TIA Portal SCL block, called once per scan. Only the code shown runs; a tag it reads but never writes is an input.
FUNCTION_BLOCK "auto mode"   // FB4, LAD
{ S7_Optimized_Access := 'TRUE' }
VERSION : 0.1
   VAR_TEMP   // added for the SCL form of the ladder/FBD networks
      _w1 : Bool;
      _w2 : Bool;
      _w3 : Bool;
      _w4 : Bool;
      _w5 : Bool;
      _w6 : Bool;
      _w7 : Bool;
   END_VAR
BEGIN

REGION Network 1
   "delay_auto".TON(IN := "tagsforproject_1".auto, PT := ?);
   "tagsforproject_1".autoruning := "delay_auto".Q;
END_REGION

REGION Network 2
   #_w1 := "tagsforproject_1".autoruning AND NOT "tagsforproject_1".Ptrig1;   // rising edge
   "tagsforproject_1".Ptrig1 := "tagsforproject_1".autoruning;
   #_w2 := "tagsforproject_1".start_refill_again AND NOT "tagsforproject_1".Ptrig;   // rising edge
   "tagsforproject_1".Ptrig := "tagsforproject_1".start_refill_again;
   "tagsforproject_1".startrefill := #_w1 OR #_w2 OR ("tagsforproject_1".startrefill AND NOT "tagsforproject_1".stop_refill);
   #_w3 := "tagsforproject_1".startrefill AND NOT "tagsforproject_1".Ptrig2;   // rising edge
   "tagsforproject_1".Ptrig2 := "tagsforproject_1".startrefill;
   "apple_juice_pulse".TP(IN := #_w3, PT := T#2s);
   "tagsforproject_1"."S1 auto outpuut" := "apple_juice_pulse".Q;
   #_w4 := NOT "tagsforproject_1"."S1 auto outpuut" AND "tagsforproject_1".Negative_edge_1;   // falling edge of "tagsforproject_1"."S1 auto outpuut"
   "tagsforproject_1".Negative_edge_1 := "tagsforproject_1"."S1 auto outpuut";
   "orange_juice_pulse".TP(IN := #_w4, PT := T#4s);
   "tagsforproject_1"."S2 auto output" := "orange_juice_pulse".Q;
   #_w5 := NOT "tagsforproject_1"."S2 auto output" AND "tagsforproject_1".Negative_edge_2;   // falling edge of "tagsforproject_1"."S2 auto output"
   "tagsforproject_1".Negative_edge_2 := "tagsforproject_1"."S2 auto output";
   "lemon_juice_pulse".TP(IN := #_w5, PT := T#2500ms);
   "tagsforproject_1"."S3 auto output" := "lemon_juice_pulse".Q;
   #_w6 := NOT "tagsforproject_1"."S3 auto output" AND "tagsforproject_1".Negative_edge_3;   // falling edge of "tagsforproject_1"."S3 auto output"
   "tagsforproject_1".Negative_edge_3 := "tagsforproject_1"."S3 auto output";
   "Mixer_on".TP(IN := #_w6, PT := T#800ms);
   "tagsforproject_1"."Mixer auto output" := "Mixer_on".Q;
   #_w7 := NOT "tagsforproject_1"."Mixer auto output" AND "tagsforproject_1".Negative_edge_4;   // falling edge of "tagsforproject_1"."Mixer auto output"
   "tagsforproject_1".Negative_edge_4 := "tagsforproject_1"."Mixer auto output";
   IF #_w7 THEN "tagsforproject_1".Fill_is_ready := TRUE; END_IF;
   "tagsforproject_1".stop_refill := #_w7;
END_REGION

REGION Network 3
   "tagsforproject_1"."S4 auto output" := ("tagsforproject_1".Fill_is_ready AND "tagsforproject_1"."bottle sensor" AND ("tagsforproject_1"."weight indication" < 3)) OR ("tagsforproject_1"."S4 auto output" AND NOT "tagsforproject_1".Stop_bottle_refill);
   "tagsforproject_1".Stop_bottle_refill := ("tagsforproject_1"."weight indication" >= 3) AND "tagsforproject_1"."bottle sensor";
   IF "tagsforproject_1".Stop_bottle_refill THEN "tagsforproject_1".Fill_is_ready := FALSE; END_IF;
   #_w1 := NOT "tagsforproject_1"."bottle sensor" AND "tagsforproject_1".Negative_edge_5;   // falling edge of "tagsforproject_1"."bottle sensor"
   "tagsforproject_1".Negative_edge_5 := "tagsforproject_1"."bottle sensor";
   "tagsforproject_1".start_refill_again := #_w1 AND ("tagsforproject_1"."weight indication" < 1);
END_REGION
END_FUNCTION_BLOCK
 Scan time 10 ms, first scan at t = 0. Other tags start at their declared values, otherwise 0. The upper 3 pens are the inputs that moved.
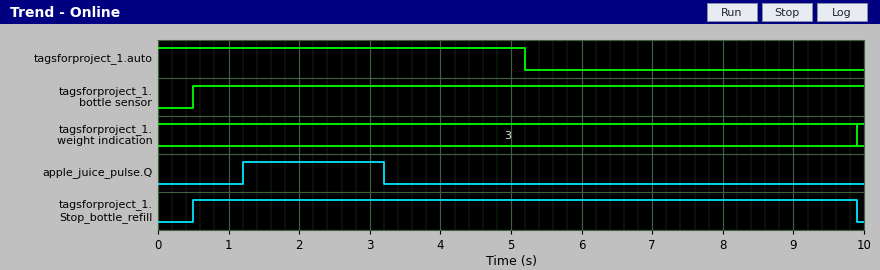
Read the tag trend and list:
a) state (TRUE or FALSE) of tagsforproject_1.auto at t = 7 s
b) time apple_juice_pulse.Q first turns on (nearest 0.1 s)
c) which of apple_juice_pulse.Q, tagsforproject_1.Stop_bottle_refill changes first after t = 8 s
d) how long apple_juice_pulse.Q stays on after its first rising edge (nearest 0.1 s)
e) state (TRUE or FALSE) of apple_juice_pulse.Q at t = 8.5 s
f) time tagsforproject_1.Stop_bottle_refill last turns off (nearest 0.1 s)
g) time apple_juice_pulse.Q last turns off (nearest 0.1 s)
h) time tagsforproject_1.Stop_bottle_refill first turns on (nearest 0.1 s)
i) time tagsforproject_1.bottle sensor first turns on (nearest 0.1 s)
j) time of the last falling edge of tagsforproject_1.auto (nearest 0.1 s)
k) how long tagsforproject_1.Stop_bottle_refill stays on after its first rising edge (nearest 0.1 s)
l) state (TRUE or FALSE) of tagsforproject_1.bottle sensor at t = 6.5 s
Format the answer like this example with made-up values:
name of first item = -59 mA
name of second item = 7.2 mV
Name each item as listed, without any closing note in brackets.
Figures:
state (TRUE or FALSE) of tagsforproject_1.auto at t = 7 s = FALSE
time apple_juice_pulse.Q first turns on = 1.2 s
which of apple_juice_pulse.Q, tagsforproject_1.Stop_bottle_refill changes first after t = 8 s = tagsforproject_1.Stop_bottle_refill
how long apple_juice_pulse.Q stays on after its first rising edge = 2.0 s
state (TRUE or FALSE) of apple_juice_pulse.Q at t = 8.5 s = FALSE
time tagsforproject_1.Stop_bottle_refill last turns off = 9.9 s
time apple_juice_pulse.Q last turns off = 3.2 s
time tagsforproject_1.Stop_bottle_refill first turns on = 0.5 s
time tagsforproject_1.bottle sensor first turns on = 0.5 s
time of the last falling edge of tagsforproject_1.auto = 5.2 s
how long tagsforproject_1.Stop_bottle_refill stays on after its first rising edge = 9.4 s
state (TRUE or FALSE) of tagsforproject_1.bottle sensor at t = 6.5 s = TRUE
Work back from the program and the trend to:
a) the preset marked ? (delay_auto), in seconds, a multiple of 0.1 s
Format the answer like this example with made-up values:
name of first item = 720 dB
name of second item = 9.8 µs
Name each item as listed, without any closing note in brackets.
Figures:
the preset marked ? (delay_auto), in seconds, a multiple of 0.1 s = 1.2 s
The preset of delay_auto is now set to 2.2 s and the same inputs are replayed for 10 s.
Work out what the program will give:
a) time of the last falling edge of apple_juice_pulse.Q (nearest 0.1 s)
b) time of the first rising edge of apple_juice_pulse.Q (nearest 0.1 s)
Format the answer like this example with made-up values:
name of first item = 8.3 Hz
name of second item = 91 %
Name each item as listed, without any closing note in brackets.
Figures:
time of the last falling edge of apple_juice_pulse.Q = 4.2 s
time of the first rising edge of apple_juice_pulse.Q = 2.2 s
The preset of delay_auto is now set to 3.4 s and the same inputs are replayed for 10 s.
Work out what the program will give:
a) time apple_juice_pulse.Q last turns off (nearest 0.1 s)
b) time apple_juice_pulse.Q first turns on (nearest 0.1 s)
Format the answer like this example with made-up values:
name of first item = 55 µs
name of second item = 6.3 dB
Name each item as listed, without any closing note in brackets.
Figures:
time apple_juice_pulse.Q last turns off = 5.4 s
time apple_juice_pulse.Q first turns on = 3.4 s
